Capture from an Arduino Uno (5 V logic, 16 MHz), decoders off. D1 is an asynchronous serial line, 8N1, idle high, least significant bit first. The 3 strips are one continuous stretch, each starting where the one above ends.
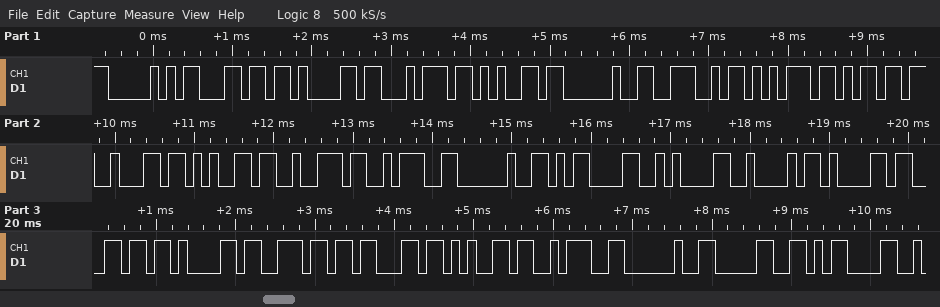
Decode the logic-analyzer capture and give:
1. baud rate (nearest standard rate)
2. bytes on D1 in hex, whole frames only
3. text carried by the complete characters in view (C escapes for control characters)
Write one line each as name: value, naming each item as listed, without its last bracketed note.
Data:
baud rate: 9600 baud
bytes on D1 in hex, whole frames only: 50 6C 61 74 65 20 4E 75 6D 62 65 72 3A 20 0D 0A 42 61 6C 61 6E 63 65 3A 20 30 0D
text carried by the complete characters in view: "Plate Number: \r\nBalance: 0\r"
